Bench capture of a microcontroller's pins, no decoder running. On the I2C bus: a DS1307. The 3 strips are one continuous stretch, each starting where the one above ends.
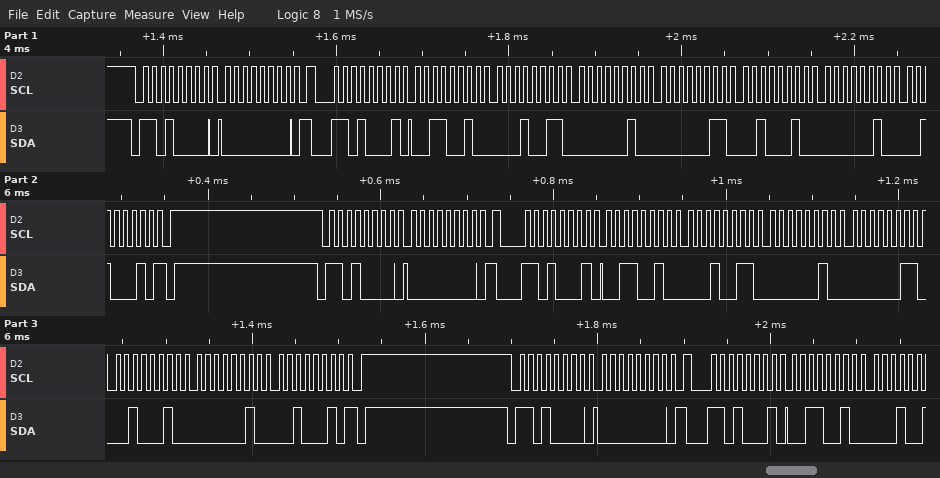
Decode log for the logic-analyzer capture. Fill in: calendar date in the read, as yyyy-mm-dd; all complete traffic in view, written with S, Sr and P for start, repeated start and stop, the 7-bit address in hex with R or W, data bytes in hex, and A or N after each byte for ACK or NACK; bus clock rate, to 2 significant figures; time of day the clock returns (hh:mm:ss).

2022-02-22
S 68W A 00 A Sr 68R A 32 A 13 A 02 A 03 A 22 A 02 A 22 N P S 68W A 00 A Sr 68R A 32 A 13 A 02 A 03 A 22 A 02 A 22 N P S 68W A 00 A Sr 68R A 32 A
100 kHz
02:13:32
